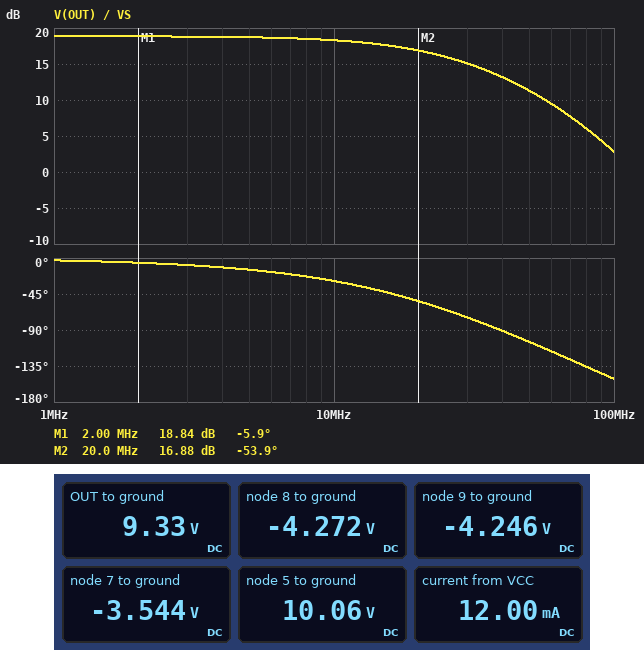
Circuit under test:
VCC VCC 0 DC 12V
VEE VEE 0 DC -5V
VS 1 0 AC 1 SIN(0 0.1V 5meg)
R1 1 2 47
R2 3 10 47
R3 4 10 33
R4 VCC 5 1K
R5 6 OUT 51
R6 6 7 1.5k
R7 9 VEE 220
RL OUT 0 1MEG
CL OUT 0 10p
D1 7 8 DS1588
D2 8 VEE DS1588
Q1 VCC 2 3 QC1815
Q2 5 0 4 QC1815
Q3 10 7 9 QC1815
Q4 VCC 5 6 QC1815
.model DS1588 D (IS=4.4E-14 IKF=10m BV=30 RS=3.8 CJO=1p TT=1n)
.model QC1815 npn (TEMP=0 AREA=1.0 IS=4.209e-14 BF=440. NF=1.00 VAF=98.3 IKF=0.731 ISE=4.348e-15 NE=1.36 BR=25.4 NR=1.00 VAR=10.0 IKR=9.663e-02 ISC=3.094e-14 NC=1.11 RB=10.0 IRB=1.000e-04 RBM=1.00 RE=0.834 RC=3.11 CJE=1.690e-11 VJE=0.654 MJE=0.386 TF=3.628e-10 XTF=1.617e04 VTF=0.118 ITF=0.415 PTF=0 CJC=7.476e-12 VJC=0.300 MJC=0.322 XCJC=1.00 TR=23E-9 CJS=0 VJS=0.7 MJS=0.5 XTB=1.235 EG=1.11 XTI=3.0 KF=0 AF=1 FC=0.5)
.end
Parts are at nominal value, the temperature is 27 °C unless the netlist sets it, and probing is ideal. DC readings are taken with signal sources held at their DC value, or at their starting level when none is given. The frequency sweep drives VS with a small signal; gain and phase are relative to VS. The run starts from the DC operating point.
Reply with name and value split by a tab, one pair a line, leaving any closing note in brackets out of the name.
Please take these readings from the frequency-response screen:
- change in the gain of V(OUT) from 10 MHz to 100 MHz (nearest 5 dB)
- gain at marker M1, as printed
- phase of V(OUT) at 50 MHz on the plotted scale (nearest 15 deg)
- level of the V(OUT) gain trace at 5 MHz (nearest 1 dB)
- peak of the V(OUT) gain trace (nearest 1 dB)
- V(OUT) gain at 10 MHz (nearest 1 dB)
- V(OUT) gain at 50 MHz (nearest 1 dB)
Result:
change in the gain of V(OUT) from 10 MHz to 100 MHz	-15 dB
gain at marker M1, as printed	18.84 dB
phase of V(OUT) at 50 MHz on the plotted scale	-105 deg
level of the V(OUT) gain trace at 5 MHz	19 dB
peak of the V(OUT) gain trace	19 dB
V(OUT) gain at 10 MHz	18 dB
V(OUT) gain at 50 MHz	11 dB
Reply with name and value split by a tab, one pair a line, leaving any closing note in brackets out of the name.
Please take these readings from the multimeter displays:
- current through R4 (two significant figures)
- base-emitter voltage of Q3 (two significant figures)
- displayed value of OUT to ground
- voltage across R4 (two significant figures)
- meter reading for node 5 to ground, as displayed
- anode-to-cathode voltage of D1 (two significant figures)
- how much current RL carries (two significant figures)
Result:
current through R4	1.9 mA
base-emitter voltage of Q3	700 mV
displayed value of OUT to ground	9.33 V
voltage across R4	1.9 V
meter reading for node 5 to ground, as displayed	10.06 V
anode-to-cathode voltage of D1	730 mV
how much current RL carries	9.3 µA
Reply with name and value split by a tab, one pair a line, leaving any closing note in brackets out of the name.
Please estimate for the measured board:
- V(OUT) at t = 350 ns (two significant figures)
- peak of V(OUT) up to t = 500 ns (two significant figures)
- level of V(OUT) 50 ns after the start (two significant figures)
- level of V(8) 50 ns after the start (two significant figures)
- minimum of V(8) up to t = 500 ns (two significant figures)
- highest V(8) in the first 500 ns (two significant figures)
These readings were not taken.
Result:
V(OUT) at t = 350 ns	8.5 V
peak of V(OUT) up to t = 500 ns	10 V
level of V(OUT) 50 ns after the start	10 V
level of V(8) 50 ns after the start	-4.3 V
minimum of V(8) up to t = 500 ns	-4.3 V
highest V(8) in the first 500 ns	-4.3 V
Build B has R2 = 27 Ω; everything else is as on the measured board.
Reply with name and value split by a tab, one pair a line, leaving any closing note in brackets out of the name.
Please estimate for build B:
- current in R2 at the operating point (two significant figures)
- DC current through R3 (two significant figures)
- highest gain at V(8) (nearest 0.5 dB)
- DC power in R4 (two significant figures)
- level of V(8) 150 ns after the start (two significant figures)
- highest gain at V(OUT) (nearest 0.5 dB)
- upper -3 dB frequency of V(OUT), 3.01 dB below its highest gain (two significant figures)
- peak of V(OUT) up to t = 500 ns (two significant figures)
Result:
current in R2 at the operating point	1.8 mA
DC current through R3	1.6 mA
highest gain at V(8)	-25.0 dB
DC power in R4	2.6 mW
level of V(8) 150 ns after the start	-4.3 V
highest gain at V(OUT)	20.5 dB
upper -3 dB frequency of V(OUT), 3.01 dB below its highest gain	25 MHz
peak of V(OUT) up to t = 500 ns	11 V
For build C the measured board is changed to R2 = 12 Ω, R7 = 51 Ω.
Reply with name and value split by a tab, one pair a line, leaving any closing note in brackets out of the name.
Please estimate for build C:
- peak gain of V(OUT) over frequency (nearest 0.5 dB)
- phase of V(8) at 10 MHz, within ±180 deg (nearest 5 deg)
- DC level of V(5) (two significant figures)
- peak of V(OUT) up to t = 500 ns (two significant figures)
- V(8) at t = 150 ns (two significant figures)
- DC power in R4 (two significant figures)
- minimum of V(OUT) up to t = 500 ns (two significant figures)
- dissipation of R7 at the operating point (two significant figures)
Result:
peak gain of V(OUT) over frequency	24.5 dB
phase of V(8) at 10 MHz, within ±180 deg	-25 deg
DC level of V(5)	7.9 V
peak of V(OUT) up to t = 500 ns	8.8 V
V(8) at t = 150 ns	-4.3 V
DC power in R4	17 mW
minimum of V(OUT) up to t = 500 ns	5.5 V
dissipation of R7 at the operating point	9.3 mW
